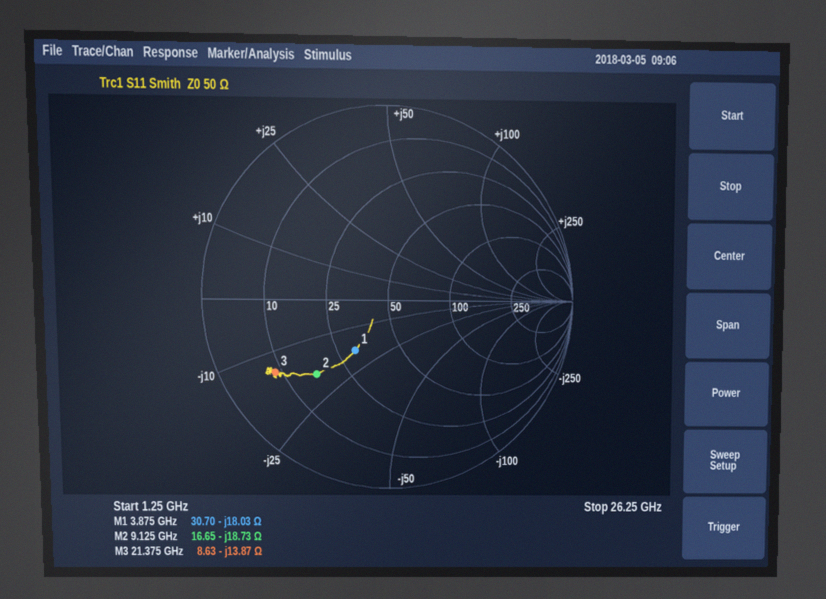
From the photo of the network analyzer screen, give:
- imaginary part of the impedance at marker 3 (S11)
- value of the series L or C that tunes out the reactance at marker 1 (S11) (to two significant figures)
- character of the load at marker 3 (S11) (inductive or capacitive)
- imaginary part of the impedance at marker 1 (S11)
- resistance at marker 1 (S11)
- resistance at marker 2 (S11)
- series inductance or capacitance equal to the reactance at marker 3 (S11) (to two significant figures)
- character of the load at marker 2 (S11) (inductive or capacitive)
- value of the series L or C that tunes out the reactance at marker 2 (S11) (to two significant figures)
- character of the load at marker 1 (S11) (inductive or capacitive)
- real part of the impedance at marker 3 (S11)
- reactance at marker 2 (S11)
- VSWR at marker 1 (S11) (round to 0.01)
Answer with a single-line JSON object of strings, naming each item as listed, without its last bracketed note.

{"imaginary part of the impedance at marker 3": "-13.87 Ω", "value of the series L or C that tunes out the reactance at marker 1 (S11)": "740 pH", "character of the load at marker 3 (S11)": "capacitive", "imaginary part of the impedance at marker 1": "-18.03 Ω", "resistance at marker 1": "30.70 Ω", "resistance at marker 2": "16.65 Ω", "series inductance or capacitance equal to the reactance at marker 3 (S11)": "540 fF", "character of the load at marker 2 (S11)": "capacitive", "value of the series L or C that tunes out the reactance at marker 2 (S11)": "330 pH", "character of the load at marker 1 (S11)": "capacitive", "real part of the impedance at marker 3": "8.63 Ω", "reactance at marker 2": "-18.73 Ω", "VSWR at marker 1 (S11)": "1.94"}
